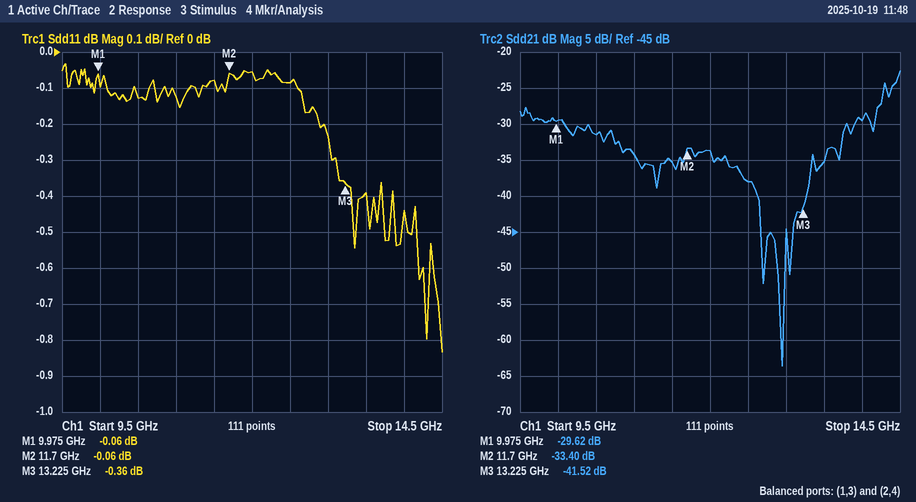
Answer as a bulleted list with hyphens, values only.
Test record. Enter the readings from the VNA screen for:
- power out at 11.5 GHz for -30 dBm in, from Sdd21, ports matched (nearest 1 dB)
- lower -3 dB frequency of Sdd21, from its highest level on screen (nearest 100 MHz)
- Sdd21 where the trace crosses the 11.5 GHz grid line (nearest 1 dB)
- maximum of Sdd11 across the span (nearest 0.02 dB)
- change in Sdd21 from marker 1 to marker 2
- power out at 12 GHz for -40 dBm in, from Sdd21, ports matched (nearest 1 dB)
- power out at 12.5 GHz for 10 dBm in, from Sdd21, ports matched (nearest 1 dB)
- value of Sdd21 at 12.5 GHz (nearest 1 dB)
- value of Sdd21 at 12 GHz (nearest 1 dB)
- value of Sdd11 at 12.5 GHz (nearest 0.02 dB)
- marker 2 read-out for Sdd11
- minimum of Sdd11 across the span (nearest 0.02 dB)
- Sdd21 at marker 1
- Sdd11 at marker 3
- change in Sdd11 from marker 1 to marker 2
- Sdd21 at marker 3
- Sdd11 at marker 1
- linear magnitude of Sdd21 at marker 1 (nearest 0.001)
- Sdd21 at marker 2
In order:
- -65 dBm
- 14.4 GHz
- -35 dB
- -0.04 dB
- -3.78 dB
- -74 dBm
- -28 dBm
- -38 dB
- -34 dB
- -0.08 dB
- -0.06 dB
- -0.84 dB
- -29.62 dB
- -0.36 dB
- 0.00 dB
- -41.52 dB
- -0.06 dB
- 0.033
- -33.40 dB
